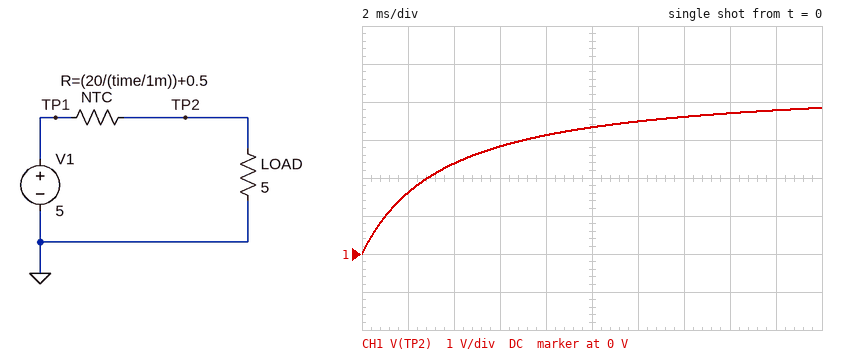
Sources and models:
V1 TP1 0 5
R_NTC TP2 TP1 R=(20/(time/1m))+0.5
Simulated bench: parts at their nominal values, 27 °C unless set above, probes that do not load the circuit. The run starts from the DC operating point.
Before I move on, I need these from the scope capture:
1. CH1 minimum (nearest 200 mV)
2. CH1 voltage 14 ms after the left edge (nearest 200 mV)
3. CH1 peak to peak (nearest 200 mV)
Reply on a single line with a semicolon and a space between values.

0 V; 3.6 V; 3.8 V
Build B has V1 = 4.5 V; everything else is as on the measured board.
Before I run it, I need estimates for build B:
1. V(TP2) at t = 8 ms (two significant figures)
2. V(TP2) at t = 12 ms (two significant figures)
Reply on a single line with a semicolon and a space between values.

2.8 V; 3.1 V
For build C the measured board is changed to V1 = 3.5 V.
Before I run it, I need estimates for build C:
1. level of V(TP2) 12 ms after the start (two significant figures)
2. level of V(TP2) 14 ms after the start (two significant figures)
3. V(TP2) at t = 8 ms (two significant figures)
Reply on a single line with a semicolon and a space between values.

2.4 V; 2.5 V; 2.2 V
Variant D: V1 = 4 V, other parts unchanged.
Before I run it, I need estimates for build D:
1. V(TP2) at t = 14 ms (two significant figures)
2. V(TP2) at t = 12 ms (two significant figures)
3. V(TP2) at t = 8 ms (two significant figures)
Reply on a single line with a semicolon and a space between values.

2.9 V; 2.8 V; 2.5 V
